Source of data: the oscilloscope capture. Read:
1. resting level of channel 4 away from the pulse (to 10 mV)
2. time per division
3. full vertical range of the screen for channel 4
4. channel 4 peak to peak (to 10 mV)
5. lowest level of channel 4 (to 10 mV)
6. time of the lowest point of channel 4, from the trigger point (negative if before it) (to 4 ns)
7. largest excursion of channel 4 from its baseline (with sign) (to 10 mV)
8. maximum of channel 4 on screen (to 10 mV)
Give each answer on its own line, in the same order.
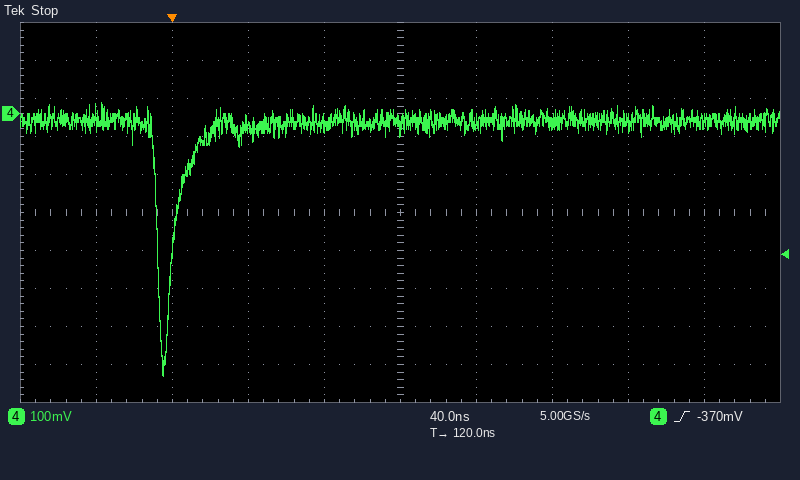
-20 mV
40 ns
1 V
720 mV
-690 mV
-4 ns
-670 mV
30 mV
